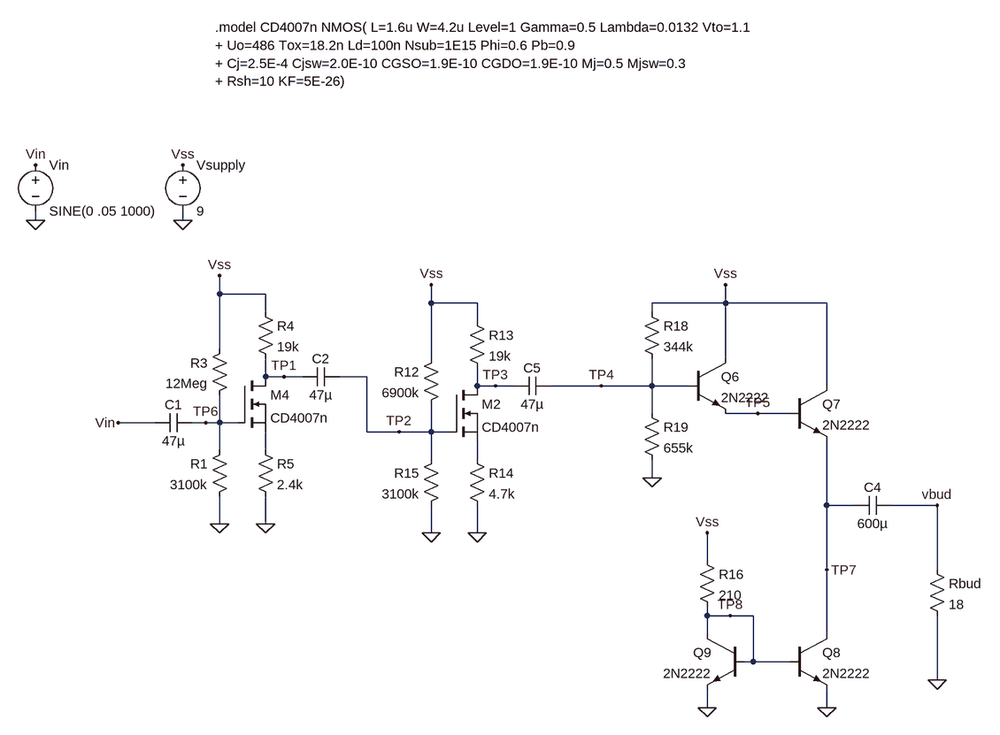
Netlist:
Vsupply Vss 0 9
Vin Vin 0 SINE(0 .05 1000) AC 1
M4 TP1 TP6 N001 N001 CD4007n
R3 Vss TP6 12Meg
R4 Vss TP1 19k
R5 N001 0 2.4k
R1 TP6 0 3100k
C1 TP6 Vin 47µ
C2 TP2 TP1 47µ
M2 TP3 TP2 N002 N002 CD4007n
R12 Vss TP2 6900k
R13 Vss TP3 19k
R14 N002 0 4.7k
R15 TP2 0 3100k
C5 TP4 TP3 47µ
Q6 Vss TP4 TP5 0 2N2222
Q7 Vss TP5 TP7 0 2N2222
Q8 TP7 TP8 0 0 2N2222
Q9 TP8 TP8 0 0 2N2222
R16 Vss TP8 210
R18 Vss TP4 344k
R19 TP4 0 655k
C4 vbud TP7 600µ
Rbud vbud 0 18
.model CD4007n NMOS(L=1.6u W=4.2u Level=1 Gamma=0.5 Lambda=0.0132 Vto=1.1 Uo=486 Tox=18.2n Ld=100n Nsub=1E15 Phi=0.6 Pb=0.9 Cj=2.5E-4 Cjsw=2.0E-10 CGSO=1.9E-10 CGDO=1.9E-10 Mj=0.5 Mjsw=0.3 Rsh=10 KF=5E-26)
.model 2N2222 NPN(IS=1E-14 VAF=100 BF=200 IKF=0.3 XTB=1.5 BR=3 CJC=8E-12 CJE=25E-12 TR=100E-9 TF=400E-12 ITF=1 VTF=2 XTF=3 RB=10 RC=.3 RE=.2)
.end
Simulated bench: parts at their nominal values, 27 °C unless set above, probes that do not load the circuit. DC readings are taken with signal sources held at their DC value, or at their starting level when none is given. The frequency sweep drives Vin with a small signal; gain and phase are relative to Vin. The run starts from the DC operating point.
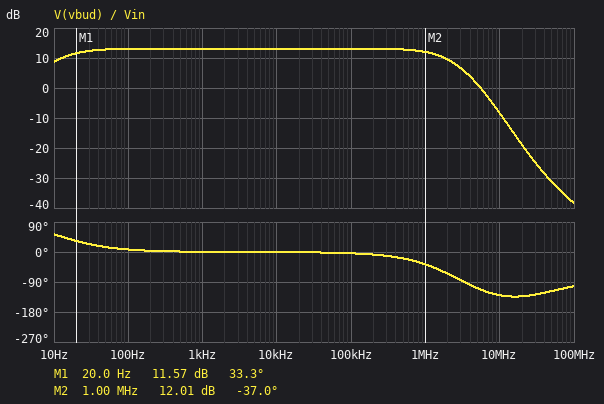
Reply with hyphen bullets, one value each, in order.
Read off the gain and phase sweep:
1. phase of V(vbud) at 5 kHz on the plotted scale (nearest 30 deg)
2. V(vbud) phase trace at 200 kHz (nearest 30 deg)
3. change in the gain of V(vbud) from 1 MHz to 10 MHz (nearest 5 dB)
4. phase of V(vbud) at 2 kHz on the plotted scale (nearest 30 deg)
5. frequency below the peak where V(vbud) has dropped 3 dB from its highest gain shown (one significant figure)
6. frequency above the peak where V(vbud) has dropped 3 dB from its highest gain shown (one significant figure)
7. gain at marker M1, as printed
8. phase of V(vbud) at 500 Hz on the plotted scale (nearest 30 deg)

- 0 deg
- 0 deg
- -20 dB
- 0 deg
- 10 Hz
- 2 MHz
- 11.57 dB
- 0 deg
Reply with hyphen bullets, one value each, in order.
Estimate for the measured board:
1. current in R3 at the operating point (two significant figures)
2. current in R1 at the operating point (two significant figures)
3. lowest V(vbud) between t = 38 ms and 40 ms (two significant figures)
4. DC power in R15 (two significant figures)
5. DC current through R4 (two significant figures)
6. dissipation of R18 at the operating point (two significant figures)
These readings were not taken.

- 600 nA
- 600 nA
- -220 mV
- 2.5 µW
- 57 µA
- 32 µW
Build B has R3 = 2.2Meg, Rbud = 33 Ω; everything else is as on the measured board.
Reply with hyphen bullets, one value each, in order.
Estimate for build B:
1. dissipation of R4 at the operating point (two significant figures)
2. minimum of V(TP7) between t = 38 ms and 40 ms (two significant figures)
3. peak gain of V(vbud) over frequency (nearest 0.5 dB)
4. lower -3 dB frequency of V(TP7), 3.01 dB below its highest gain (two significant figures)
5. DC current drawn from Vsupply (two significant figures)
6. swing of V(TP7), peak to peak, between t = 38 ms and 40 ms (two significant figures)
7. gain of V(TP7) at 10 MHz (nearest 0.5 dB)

- 3.0 mW
- 4.3 V
- -11.0 dB
- 15 mHz
- 80 mA
- 29 mV
- -30.0 dB
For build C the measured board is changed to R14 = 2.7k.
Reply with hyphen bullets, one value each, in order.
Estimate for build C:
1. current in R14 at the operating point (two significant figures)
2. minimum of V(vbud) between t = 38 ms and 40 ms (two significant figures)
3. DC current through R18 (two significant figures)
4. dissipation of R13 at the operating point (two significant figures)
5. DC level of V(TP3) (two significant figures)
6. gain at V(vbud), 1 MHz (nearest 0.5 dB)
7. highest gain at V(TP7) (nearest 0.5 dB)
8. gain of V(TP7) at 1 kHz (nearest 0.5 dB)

- 200 µA
- -320 mV
- 9.7 µA
- 730 µW
- 5.3 V
- 15.0 dB
- 17.0 dB
- 16.0 dB
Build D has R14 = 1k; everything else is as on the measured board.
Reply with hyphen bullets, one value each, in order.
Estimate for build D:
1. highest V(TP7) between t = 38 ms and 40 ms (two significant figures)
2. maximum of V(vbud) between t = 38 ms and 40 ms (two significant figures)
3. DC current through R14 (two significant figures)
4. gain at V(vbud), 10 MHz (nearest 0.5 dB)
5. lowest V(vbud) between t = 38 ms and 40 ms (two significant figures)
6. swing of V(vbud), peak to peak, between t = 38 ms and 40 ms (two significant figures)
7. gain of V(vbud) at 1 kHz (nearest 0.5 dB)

- 4.8 V
- 510 mV
- 280 µA
- -1.0 dB
- -500 mV
- 1.0 V
- 20.0 dB
